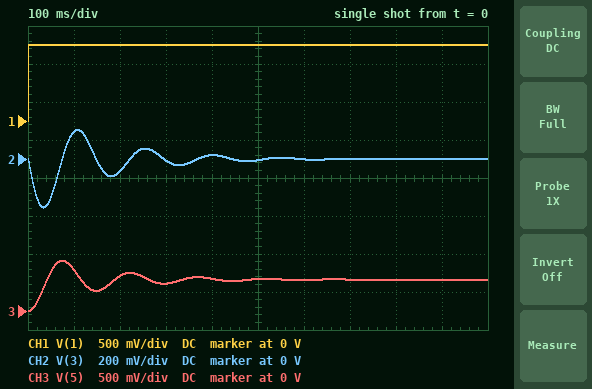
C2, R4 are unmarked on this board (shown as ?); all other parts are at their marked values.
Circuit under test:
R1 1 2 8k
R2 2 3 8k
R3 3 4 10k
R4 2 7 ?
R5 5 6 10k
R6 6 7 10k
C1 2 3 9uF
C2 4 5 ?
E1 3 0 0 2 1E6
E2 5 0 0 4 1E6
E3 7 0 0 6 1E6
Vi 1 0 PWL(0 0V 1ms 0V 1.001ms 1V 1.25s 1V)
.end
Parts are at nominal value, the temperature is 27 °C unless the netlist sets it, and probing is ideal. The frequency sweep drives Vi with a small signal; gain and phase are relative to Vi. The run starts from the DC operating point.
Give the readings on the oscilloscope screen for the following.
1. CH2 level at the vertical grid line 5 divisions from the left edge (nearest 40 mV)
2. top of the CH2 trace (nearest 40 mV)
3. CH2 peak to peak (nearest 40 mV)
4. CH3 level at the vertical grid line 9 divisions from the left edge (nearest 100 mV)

0 V
160 mV
400 mV
400 mV
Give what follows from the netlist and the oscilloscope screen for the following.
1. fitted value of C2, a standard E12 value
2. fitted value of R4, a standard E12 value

1.8 µF
3.3 kΩ
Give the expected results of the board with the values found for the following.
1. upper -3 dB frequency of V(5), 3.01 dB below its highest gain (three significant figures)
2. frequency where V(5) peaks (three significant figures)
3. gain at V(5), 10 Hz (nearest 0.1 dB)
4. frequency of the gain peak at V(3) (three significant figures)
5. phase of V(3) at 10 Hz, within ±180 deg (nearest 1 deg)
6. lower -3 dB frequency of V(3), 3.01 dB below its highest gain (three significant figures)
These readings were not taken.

7.74 Hz
6.70 Hz
-9.3 dB
6.88 Hz
113 deg
5.87 Hz
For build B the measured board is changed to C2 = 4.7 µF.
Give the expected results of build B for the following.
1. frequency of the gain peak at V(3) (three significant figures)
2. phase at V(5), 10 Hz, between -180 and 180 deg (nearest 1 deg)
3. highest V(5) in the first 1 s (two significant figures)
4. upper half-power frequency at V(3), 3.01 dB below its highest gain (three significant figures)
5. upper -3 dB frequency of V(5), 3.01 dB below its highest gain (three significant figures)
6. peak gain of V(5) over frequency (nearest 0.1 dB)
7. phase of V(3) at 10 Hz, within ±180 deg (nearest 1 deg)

4.26 Hz
-165 deg
590 mV
5.51 Hz
4.98 Hz
-1.7 dB
105 deg
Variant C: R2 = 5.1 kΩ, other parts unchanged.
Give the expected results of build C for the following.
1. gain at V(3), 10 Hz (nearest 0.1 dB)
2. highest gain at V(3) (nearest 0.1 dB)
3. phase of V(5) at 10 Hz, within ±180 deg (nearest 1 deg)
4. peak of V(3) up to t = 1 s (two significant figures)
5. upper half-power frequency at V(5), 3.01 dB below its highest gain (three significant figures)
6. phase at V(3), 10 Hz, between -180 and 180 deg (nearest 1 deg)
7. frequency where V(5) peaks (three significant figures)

-9.1 dB
-3.9 dB
-147 deg
100 mV
8.03 Hz
123 deg
6.43 Hz
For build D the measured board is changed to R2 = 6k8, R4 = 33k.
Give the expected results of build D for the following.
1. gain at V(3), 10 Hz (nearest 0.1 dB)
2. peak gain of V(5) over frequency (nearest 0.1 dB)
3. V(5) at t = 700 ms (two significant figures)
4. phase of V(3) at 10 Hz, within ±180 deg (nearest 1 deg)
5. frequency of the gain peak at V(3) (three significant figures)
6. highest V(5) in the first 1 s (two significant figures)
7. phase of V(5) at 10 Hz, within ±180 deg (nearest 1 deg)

-13.0 dB
12.7 dB
4.1 V
105 deg
2.18 Hz
4.5 V
-165 deg
